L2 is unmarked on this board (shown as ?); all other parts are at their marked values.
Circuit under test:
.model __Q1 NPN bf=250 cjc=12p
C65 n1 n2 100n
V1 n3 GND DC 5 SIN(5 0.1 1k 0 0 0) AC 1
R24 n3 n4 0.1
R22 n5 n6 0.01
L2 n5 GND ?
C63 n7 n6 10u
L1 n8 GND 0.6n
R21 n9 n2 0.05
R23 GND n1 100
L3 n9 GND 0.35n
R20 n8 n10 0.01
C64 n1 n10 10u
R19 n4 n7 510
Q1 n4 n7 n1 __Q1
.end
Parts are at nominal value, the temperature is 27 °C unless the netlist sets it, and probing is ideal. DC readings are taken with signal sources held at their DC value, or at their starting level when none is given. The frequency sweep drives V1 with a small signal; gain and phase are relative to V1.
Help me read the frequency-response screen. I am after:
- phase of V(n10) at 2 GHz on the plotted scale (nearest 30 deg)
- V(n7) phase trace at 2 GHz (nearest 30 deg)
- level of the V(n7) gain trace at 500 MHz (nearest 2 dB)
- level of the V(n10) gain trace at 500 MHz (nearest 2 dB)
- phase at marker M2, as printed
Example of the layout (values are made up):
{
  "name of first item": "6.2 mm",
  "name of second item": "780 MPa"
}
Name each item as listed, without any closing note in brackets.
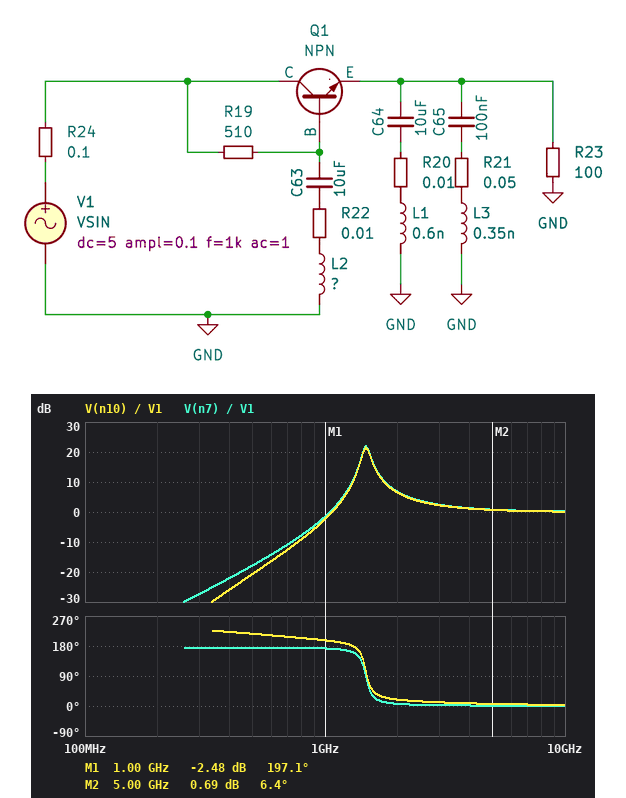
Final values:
{
  "phase of V(n10) at 2 GHz on the plotted scale": "30 deg",
  "V(n7) phase trace at 2 GHz": "0 deg",
  "level of the V(n7) gain trace at 500 MHz": "-18 dB",
  "level of the V(n10) gain trace at 500 MHz": "-20 dB",
  "phase at marker M2, as printed": "6.4 deg"
}
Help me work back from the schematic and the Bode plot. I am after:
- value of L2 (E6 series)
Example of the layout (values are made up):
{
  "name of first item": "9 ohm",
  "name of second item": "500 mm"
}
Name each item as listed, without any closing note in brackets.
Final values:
{
  "value of L2": "1 nH"
}
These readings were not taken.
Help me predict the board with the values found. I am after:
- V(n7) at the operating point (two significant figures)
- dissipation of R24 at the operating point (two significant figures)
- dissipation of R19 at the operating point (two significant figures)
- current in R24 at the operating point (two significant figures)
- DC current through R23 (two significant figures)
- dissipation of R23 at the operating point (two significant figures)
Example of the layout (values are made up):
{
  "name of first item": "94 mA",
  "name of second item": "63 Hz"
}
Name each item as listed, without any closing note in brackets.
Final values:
{
  "V(n7) at the operating point": "4.9 V",
  "dissipation of R24 at the operating point": "160 µW",
  "dissipation of R19 at the operating point": "13 µW",
  "current in R24 at the operating point": "40 mA",
  "DC current through R23": "40 mA",
  "dissipation of R23 at the operating point": "160 mW"
}
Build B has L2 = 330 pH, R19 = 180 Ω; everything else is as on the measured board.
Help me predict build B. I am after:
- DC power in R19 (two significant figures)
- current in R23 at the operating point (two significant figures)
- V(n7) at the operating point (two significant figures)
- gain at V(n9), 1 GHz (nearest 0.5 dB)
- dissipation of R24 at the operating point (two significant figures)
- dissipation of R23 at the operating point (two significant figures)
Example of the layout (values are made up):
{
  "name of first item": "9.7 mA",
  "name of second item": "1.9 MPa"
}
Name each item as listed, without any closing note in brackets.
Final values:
{
  "DC power in R19": "4.8 µW",
  "current in R23 at the operating point": "41 mA",
  "V(n7) at the operating point": "5.0 V",
  "gain at V(n9), 1 GHz": "-15.5 dB",
  "dissipation of R24 at the operating point": "170 µW",
  "dissipation of R23 at the operating point": "170 mW"
}
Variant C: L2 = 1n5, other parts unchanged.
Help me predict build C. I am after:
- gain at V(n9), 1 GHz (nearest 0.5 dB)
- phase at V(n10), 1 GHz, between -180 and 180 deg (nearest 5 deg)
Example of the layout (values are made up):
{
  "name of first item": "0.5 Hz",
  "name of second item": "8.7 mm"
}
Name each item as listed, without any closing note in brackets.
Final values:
{
  "gain at V(n9), 1 GHz": "5.5 dB",
  "phase at V(n10), 1 GHz, between -180 and 180 deg": "-170 deg"
}
